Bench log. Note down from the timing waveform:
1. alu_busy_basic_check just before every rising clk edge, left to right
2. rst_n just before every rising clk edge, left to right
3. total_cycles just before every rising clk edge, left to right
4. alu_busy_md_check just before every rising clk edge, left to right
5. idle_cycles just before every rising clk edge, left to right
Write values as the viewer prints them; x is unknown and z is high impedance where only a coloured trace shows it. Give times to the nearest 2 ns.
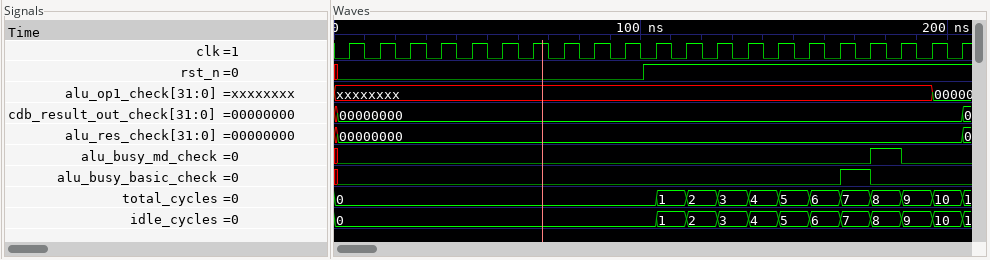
0 0 0 0 0 0 0 0 0 0 0 0 0 0 0 0 0 1 0 0 0
0 0 0 0 0 0 0 0 0 0 1 1 1 1 1 1 1 1 1 1 1
0, 0, 0, 0, 0, 0, 0, 0, 0, 0, 0, 1, 2, 3, 4, 5, 6, 7, 8, 9, 10
0 0 0 0 0 0 0 0 0 0 0 0 0 0 0 0 0 0 1 0 0
0, 0, 0, 0, 0, 0, 0, 0, 0, 0, 0, 1, 2, 3, 4, 5, 6, 7, 8, 9, 10
